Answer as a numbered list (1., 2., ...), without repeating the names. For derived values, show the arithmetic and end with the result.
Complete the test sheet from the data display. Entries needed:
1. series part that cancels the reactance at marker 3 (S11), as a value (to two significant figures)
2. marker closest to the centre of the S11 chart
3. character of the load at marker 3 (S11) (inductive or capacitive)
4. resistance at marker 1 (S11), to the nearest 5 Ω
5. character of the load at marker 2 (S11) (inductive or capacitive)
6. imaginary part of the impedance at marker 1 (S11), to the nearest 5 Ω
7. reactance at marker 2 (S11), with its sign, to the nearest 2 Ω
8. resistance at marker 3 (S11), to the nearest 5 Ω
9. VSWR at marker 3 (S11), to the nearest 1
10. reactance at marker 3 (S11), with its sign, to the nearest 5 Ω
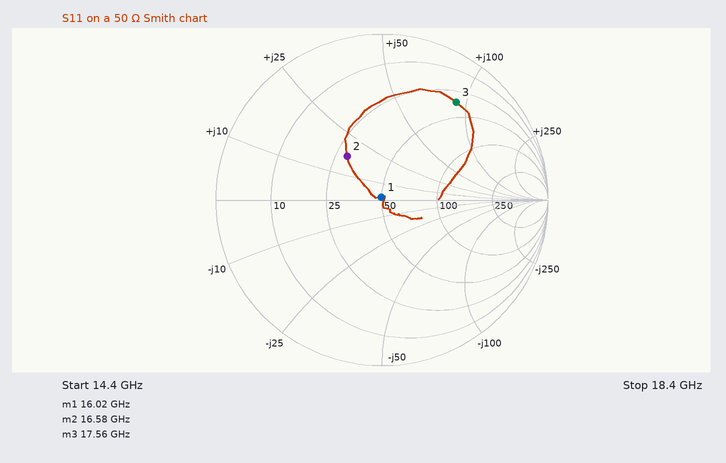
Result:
1. C = 1/(2π × 17.56 GHz × 90 Ω) ≈ 101 fF, so 100 fF to two significant figures
2. marker 1
3. inductive
4. 50 Ω
5. inductive
6. 0 Ω
7. +18 Ω
8. 35 Ω
9. 7
10. +90 Ω
